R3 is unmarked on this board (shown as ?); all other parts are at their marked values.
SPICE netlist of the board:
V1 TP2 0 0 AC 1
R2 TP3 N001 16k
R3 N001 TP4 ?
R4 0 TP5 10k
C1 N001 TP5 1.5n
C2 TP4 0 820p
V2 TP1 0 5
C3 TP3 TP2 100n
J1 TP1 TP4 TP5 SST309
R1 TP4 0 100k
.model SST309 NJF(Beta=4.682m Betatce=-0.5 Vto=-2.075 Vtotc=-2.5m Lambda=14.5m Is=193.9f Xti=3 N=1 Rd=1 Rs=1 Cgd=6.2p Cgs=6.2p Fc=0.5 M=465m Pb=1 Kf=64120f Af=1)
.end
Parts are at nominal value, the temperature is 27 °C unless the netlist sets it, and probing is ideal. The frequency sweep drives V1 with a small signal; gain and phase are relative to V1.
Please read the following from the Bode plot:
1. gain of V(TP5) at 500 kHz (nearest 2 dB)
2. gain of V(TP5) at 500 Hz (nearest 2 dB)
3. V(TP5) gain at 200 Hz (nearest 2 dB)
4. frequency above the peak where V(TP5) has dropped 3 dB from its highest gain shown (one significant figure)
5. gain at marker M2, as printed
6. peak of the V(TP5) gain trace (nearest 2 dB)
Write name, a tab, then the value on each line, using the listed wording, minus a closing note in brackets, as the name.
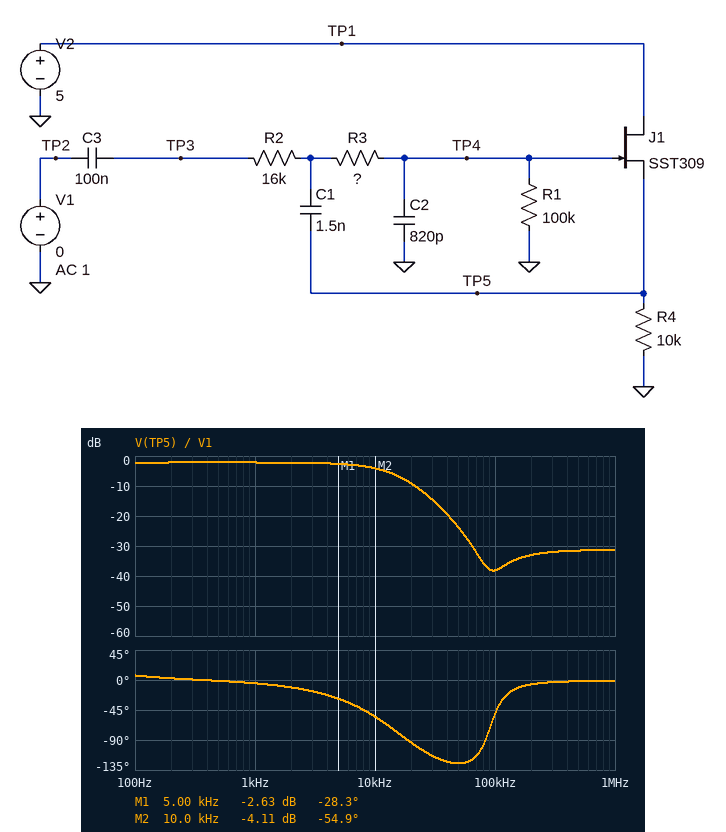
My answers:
gain of V(TP5) at 500 kHz	-32 dB
gain of V(TP5) at 500 Hz	-2 dB
V(TP5) gain at 200 Hz	-2 dB
frequency above the peak where V(TP5) has dropped 3 dB from its highest gain shown	10 kHz
gain at marker M2, as printed	-4.11 dB
peak of the V(TP5) gain trace	-2 dB
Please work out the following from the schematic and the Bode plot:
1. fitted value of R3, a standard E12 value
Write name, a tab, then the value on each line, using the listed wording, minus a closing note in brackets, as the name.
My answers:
fitted value of R3, a standard E12 value	4.7 kΩ
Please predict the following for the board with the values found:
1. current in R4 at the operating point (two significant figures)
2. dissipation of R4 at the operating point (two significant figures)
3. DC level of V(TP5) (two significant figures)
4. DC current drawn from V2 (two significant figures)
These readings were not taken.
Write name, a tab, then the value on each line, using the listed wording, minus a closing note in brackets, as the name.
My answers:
current in R4 at the operating point	190 µA
dissipation of R4 at the operating point	350 µW
DC level of V(TP5)	1.9 V
DC current drawn from V2	190 µA
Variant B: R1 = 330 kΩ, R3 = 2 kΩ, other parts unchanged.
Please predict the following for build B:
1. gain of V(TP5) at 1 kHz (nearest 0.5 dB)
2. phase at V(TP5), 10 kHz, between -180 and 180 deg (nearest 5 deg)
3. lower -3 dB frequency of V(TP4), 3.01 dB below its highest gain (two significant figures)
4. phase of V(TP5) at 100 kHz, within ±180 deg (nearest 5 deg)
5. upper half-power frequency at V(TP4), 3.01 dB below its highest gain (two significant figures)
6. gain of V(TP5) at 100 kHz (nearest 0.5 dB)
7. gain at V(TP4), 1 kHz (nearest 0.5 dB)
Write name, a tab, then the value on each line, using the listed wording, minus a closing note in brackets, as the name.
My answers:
gain of V(TP5) at 1 kHz	-1.0 dB
phase at V(TP5), 10 kHz, between -180 and 180 deg	-50 deg
lower -3 dB frequency of V(TP4), 3.01 dB below its highest gain	4.5 Hz
phase of V(TP5) at 100 kHz, within ±180 deg	-105 deg
upper half-power frequency at V(TP4), 3.01 dB below its highest gain	12 kHz
gain of V(TP5) at 100 kHz	-30.5 dB
gain at V(TP4), 1 kHz	-0.5 dB
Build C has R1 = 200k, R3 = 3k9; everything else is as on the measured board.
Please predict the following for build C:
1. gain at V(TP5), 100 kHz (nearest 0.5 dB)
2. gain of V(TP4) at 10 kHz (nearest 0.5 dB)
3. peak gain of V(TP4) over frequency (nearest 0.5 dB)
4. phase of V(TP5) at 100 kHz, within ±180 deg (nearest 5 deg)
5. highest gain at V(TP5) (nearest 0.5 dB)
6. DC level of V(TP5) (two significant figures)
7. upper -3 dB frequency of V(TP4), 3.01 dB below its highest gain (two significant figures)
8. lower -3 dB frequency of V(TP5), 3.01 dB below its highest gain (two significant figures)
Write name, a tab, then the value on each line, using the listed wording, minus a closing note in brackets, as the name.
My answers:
gain at V(TP5), 100 kHz	-37.5 dB
gain of V(TP4) at 10 kHz	-3.0 dB
peak gain of V(TP4) over frequency	-1.0 dB
phase of V(TP5) at 100 kHz, within ±180 deg	-70 deg
highest gain at V(TP5)	-1.5 dB
DC level of V(TP5)	1.9 V
upper -3 dB frequency of V(TP4), 3.01 dB below its highest gain	12 kHz
lower -3 dB frequency of V(TP5), 3.01 dB below its highest gain	7.2 Hz
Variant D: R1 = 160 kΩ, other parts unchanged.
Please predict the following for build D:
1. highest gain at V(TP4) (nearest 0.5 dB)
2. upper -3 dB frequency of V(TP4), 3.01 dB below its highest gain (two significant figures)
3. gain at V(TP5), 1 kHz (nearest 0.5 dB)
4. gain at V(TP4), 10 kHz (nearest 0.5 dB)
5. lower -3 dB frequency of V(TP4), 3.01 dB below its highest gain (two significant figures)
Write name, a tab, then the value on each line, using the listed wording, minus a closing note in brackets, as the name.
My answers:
highest gain at V(TP4)	-1.0 dB
upper -3 dB frequency of V(TP4), 3.01 dB below its highest gain	12 kHz
gain at V(TP5), 1 kHz	-1.5 dB
gain at V(TP4), 10 kHz	-3.0 dB
lower -3 dB frequency of V(TP4), 3.01 dB below its highest gain	8.7 Hz
